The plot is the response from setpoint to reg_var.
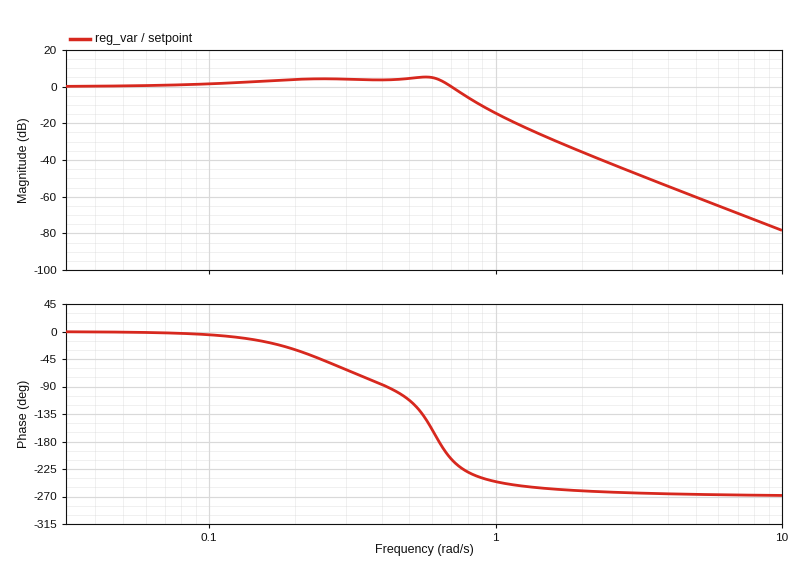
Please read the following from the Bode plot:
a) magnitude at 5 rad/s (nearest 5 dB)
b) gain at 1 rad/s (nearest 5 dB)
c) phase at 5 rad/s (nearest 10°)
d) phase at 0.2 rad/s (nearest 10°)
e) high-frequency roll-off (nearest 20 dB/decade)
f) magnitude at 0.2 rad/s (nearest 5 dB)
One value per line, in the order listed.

-60 dB
-15 dB
-270°
-30°
-60 dB/decade
5 dB
